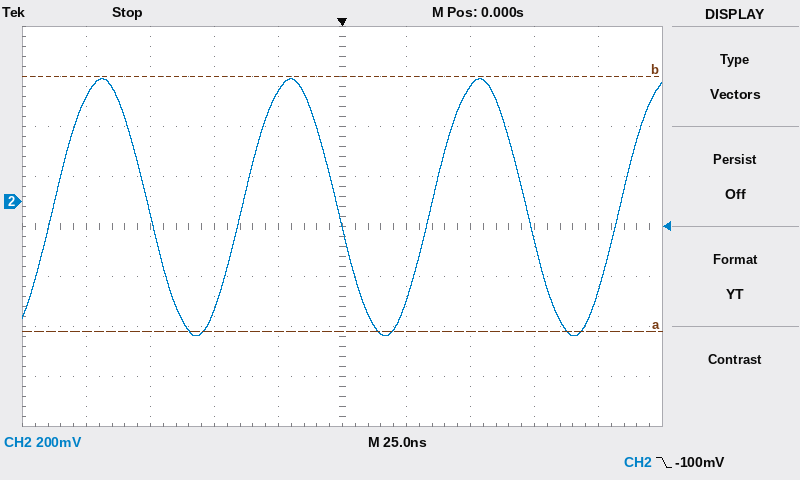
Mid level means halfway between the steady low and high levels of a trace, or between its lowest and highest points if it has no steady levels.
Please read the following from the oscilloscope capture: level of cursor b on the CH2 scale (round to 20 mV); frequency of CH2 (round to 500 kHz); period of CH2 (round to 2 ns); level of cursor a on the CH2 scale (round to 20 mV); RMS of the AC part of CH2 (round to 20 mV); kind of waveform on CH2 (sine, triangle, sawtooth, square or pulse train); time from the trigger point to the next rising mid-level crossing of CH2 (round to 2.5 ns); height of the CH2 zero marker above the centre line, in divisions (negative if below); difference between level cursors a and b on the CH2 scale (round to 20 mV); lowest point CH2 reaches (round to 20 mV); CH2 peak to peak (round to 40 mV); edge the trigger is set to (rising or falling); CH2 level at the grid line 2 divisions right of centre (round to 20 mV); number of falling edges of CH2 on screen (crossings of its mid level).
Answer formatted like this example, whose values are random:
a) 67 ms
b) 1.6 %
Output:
a) 500 mV
b) 13.5 MHz
c) 74 ns
d) -520 mV
e) 360 mV
f) sine
g) 35.0 ns
h) +0.5 div
i) 1.02 V
j) -540 mV
k) 1.04 V
l) falling
m) 460 mV
n) 3
